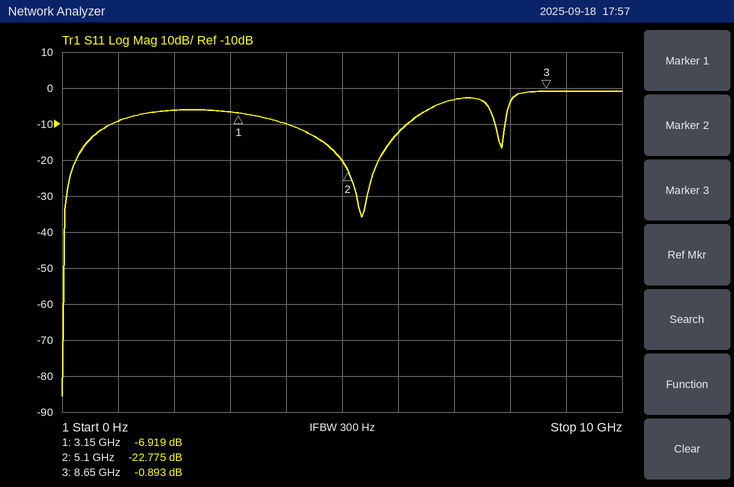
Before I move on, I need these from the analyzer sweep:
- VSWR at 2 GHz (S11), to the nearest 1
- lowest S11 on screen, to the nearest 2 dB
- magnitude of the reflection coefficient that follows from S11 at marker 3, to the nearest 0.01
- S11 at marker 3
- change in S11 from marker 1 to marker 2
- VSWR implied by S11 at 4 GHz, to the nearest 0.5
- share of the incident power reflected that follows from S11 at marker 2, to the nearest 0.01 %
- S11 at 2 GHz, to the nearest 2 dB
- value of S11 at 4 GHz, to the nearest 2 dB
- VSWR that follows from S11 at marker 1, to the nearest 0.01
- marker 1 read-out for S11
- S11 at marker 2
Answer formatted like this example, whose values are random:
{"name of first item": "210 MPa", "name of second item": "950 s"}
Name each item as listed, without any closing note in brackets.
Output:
{"VSWR at 2 GHz (S11), to the nearest 1": "3", "lowest S11 on screen, to the nearest 2 dB": "-86 dB", "magnitude of the reflection coefficient that follows from S11 at marker 3, to the nearest 0.01": "0.90", "S11 at marker 3": "-0.893 dB", "change in S11 from marker 1 to marker 2": "-15.856 dB", "VSWR implied by S11 at 4 GHz, to the nearest 0.5": "2.0", "share of the incident power reflected that follows from S11 at marker 2, to the nearest 0.01 %": "0.53 %", "S11 at 2 GHz, to the nearest 2 dB": "-6 dB", "value of S11 at 4 GHz, to the nearest 2 dB": "-10 dB", "VSWR that follows from S11 at marker 1, to the nearest 0.01": "2.64", "marker 1 read-out for S11": "-6.919 dB", "S11 at marker 2": "-22.775 dB"}
